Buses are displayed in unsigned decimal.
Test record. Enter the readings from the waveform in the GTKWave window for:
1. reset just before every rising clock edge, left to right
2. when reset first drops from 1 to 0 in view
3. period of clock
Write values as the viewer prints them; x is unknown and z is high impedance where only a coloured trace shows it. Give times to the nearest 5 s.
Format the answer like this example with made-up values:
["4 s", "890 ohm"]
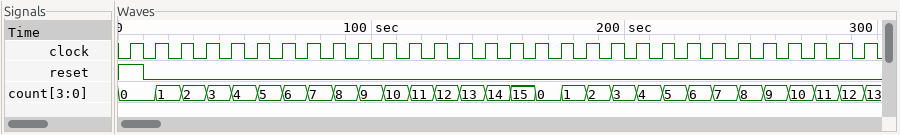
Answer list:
["1 0 0 0 0 0 0 0 0 0 0 0 0 0 0 0 0 0 0 0 0 0 0 0 0 0 0 0 0 0", "10 s", "10 s"]
